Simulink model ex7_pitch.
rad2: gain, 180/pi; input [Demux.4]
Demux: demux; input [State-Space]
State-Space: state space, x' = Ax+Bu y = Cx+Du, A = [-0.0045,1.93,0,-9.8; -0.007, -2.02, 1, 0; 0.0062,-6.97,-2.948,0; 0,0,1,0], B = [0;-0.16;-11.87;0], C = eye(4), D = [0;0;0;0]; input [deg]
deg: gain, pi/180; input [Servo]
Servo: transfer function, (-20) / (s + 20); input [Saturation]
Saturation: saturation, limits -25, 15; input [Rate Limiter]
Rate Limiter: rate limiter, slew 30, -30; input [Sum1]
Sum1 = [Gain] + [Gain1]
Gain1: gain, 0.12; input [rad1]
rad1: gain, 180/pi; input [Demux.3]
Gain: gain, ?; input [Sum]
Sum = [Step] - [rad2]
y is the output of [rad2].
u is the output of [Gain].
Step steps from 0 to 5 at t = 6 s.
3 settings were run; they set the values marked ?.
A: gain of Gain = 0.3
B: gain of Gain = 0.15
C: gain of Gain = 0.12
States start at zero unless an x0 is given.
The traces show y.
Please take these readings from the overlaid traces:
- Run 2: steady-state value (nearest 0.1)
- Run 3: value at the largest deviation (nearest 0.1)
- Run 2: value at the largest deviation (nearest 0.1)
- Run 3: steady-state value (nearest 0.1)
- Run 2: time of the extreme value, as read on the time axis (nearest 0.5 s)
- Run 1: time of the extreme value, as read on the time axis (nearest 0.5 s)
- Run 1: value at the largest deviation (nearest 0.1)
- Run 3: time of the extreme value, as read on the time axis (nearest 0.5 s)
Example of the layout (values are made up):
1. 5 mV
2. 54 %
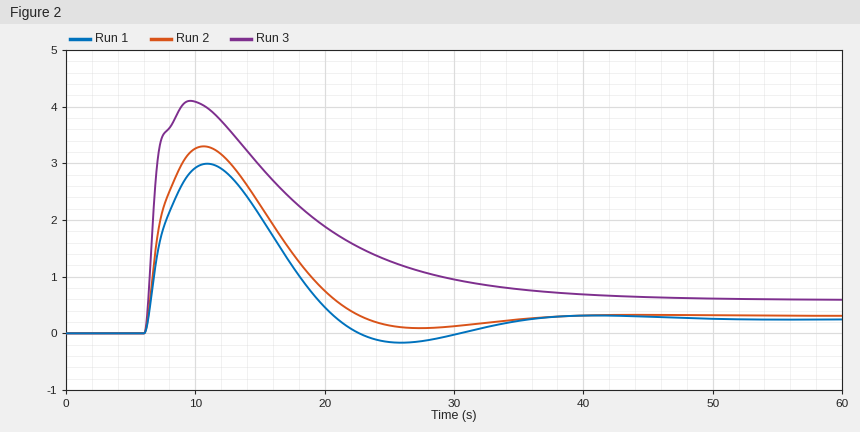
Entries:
1. 0.3
2. 4.1
3. 3.3
4. 0.6
5. 10.5 s
6. 11.0 s
7. 3.0
8. 9.5 s
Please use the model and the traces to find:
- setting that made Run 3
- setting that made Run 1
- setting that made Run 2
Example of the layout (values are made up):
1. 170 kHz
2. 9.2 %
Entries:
1. A
2. C
3. B
